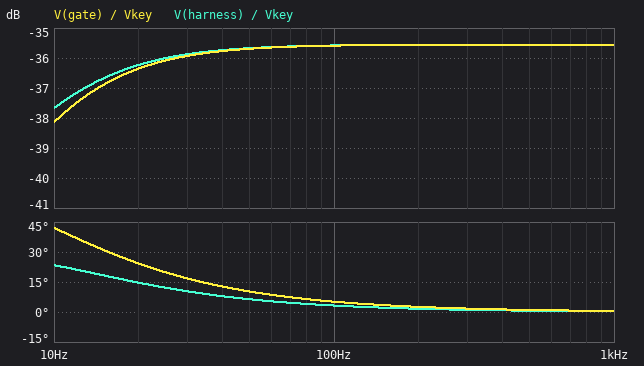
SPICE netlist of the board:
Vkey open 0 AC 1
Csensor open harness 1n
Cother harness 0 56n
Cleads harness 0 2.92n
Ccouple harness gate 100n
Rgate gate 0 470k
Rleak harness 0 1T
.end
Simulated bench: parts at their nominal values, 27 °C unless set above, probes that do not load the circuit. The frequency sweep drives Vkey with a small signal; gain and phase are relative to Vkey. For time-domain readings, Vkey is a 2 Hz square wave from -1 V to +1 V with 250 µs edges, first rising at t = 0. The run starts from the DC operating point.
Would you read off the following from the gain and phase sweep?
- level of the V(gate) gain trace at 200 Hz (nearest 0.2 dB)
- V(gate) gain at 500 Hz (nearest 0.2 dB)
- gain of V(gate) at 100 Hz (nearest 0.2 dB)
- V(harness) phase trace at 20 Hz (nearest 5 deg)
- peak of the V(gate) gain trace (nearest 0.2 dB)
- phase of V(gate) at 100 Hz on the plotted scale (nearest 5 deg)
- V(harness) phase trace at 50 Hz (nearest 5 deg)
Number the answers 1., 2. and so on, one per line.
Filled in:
1. -35.6 dB
2. -35.6 dB
3. -35.6 dB
4. 15 deg
5. -35.6 dB
6. 5 deg
7. 5 deg
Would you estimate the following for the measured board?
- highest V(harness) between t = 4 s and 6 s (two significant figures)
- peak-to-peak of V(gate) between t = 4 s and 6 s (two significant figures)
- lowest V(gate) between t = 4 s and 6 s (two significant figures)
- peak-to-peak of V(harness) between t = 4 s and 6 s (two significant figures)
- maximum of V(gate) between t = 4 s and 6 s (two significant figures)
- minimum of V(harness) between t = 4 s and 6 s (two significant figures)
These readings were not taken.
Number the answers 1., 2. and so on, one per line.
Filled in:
1. 33 mV
2. 66 mV
3. -33 mV
4. 54 mV
5. 33 mV
6. -21 mV
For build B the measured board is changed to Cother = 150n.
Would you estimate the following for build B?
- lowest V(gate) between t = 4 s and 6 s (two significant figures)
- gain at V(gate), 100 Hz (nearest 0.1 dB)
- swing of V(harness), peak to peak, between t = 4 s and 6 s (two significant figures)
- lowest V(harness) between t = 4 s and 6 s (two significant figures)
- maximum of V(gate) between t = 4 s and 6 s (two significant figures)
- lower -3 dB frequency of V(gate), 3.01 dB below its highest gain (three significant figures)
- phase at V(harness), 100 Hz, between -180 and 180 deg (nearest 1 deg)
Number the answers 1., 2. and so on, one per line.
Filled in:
1. -13 mV
2. -43.8 dB
3. 18 mV
4. -5.1 mV
5. 13 mV
6. 5.59 Hz
7. 1 deg
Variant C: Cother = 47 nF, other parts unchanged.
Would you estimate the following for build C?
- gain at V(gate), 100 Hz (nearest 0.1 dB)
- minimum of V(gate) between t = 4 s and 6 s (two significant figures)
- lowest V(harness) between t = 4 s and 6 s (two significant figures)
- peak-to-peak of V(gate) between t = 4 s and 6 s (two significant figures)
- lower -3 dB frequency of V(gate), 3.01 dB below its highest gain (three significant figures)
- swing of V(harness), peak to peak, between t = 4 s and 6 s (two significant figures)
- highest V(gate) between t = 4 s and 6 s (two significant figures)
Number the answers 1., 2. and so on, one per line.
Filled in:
1. -34.2 dB
2. -39 mV
3. -26 mV
4. 78 mV
5. 10.0 Hz
6. 65 mV
7. 39 mV
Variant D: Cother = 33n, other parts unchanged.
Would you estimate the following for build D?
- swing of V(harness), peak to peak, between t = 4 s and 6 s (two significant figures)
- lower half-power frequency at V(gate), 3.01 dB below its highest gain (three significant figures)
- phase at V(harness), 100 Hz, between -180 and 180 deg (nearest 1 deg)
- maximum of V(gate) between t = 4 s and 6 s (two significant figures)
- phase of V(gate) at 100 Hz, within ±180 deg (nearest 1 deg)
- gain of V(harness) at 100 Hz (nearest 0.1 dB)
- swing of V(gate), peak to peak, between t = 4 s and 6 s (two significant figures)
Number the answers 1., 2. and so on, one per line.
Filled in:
1. 93 mV
2. 12.6 Hz
3. 5 deg
4. 54 mV
5. 7 deg
6. -31.4 dB
7. 110 mV
